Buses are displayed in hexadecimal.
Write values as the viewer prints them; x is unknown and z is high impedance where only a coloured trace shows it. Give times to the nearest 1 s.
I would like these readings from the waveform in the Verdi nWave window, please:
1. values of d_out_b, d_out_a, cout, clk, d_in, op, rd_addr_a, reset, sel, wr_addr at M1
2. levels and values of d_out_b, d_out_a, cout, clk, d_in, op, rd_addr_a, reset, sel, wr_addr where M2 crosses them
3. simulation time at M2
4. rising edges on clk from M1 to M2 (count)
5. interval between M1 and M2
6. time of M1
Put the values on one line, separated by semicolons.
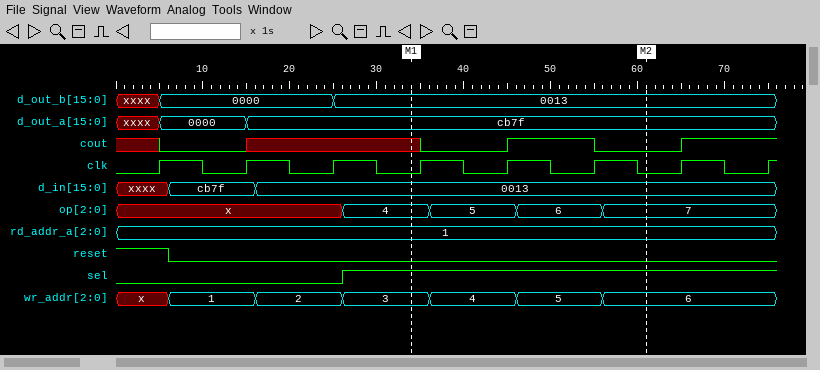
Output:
d_out_b=0013, d_out_a=cb7f, cout=x, clk=0, d_in=0013, op=4, rd_addr_a=1, reset=0, sel=1, wr_addr=3; d_out_b=0013, d_out_a=cb7f, cout=0, clk=0, d_in=0013, op=7, rd_addr_a=1, reset=0, sel=1, wr_addr=6; 61 s; 3; 27 s; 34 s
